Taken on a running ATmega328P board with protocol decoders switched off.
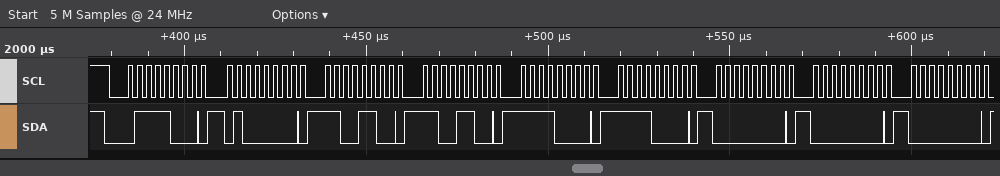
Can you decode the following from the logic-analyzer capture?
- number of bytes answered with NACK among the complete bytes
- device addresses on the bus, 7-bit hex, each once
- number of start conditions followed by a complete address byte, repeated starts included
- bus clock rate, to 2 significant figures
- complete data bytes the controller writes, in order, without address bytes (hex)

0
0x3C
1
400 kHz
40 CC CC F0 F0 00 00 00
